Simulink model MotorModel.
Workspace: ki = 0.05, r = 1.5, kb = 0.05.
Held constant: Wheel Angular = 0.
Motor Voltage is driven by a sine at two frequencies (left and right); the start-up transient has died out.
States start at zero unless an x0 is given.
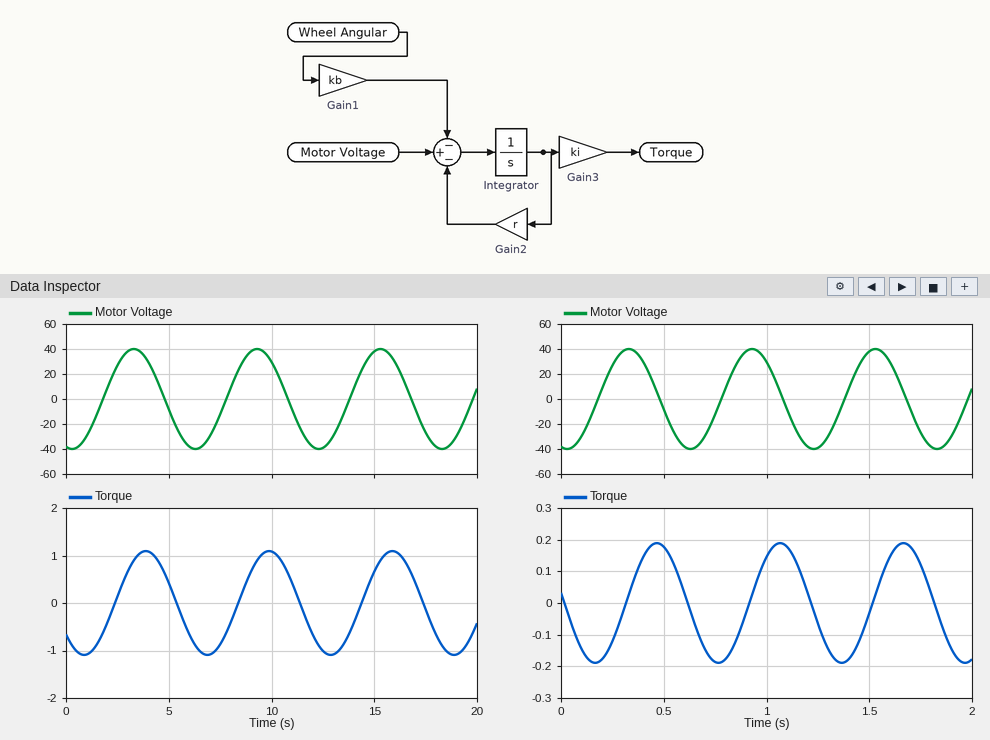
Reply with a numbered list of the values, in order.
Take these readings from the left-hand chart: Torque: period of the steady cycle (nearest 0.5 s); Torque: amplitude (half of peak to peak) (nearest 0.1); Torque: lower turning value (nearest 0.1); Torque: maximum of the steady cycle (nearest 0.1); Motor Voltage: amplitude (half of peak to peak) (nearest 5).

1. 6.0 s
2. 1.1
3. -1.1
4. 1.1
5. 40
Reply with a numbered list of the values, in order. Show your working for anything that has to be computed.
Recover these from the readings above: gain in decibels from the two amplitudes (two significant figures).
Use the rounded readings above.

1. 20 log10(1.1 / 40) = -31 dB
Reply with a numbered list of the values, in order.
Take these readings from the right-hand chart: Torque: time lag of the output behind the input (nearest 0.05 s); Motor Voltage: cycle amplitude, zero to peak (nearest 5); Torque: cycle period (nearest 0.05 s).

1. 0.15 s
2. 40
3. 0.60 s
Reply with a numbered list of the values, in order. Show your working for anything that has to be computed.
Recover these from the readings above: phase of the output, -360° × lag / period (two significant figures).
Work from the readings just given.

1. -360 × 0.15 / 0.6 = -90°
